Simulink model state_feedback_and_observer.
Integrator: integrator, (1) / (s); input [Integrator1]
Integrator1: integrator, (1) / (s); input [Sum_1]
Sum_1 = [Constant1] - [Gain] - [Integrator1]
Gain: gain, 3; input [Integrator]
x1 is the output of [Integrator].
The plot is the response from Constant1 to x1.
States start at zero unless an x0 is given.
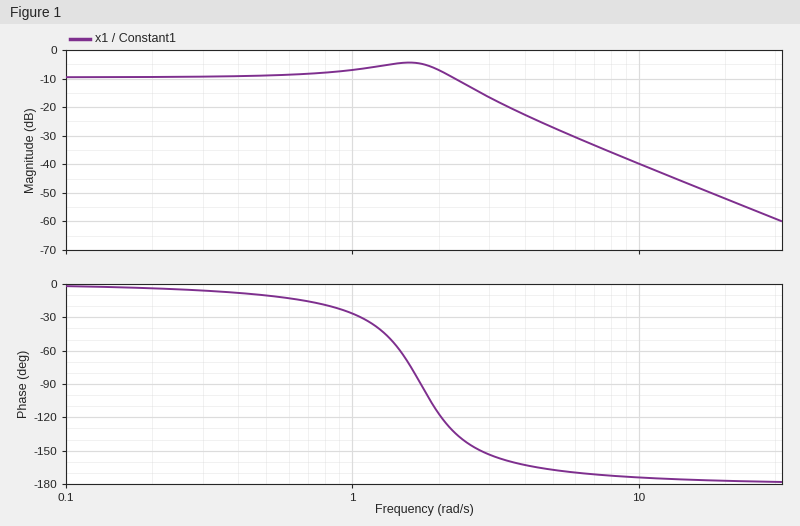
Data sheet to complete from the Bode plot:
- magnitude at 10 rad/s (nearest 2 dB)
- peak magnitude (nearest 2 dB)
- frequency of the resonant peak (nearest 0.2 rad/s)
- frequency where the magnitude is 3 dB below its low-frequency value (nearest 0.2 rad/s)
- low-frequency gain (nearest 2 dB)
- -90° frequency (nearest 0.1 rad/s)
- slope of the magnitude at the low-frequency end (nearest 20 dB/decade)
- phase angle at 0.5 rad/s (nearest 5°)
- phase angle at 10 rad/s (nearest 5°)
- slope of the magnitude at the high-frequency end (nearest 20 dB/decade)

-40 dB
-4 dB
1.6 rad/s
2.6 rad/s
-10 dB
1.7 rad/s
0 dB/decade
-10°
-175°
-40 dB/decade
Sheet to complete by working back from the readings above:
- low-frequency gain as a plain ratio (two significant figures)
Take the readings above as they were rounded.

0.32
